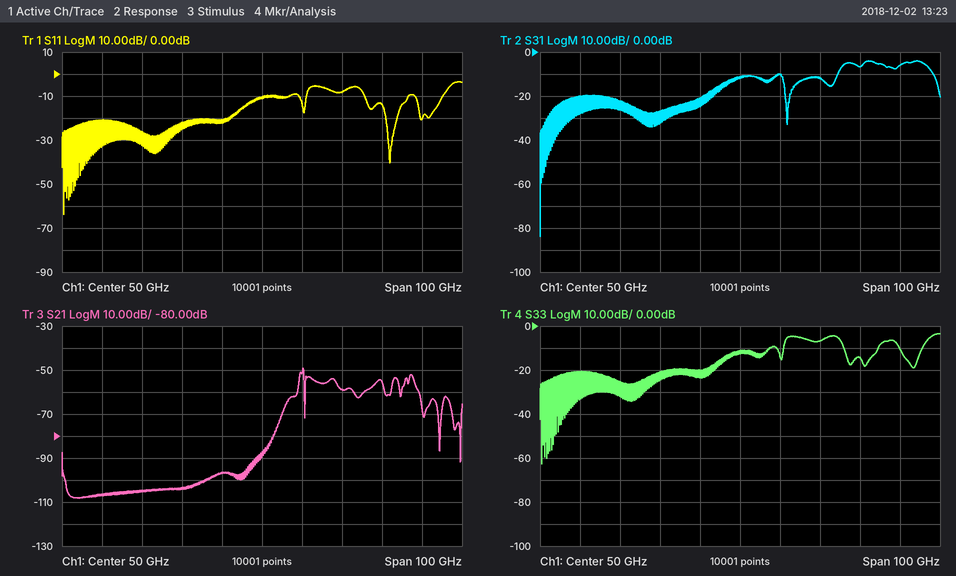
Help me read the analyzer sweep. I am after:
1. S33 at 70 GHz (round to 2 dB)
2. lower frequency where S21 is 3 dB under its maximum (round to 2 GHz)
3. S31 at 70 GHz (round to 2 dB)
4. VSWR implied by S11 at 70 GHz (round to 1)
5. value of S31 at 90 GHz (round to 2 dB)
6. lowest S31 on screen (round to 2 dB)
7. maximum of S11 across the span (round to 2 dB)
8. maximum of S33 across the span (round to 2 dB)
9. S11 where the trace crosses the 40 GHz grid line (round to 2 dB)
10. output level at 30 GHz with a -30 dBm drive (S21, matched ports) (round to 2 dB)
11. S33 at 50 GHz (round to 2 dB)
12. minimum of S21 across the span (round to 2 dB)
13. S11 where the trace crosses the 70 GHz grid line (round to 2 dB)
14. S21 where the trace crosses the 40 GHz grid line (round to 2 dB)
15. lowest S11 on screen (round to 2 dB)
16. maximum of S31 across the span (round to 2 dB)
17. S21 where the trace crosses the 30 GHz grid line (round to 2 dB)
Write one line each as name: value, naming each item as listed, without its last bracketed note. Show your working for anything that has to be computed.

S33 at 70 GHz: -6 dB
lower frequency where S21 is 3 dB under its maximum: 60 GHz
S31 at 70 GHz: -12 dB
VSWR implied by S11 at 70 GHz: |Γ| = 10^(-8/20) = 0.3981; VSWR = (1 + 0.3981)/(1 − 0.3981) ≈ 2
value of S31 at 90 GHz: -6 dB
lowest S31 on screen: -84 dB
maximum of S11 across the span: -4 dB
maximum of S33 across the span: -4 dB
S11 where the trace crosses the 40 GHz grid line: -22 dB
output level at 30 GHz with a -30 dBm drive (S21, matched ports): -30 dBm + (-104 dB) = -134 dBm
S33 at 50 GHz: -12 dB
minimum of S21 across the span: -108 dB
S11 where the trace crosses the 70 GHz grid line: -8 dB
S21 where the trace crosses the 40 GHz grid line: -96 dB
lowest S11 on screen: -64 dB
maximum of S31 across the span: -4 dB
S21 where the trace crosses the 30 GHz grid line: -104 dB
